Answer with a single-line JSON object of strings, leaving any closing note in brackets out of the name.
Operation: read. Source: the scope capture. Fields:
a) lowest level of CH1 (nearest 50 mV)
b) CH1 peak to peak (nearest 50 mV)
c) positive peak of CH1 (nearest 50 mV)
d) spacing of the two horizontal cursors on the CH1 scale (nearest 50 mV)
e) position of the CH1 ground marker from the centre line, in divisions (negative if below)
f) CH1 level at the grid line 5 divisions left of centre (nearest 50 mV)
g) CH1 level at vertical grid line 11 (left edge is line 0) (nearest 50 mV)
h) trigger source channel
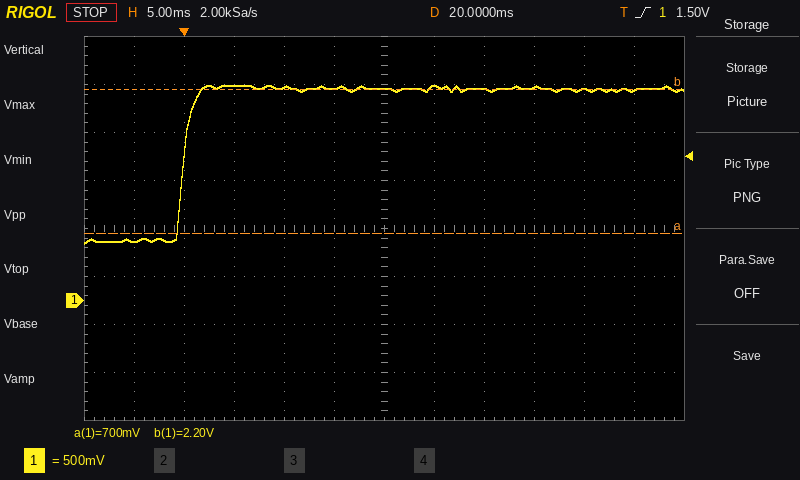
{"lowest level of CH1": "600 mV", "CH1 peak to peak": "1.65 V", "positive peak of CH1": "2.25 V", "spacing of the two horizontal cursors on the CH1 scale": "1.50 V", "position of the CH1 ground marker from the centre line, in divisions": "-1.5 div", "CH1 level at the grid line 5 divisions left of centre": "600 mV", "CH1 level at vertical grid line 11 (left edge is line 0)": "2.20 V", "trigger source channel": "CH1"}
